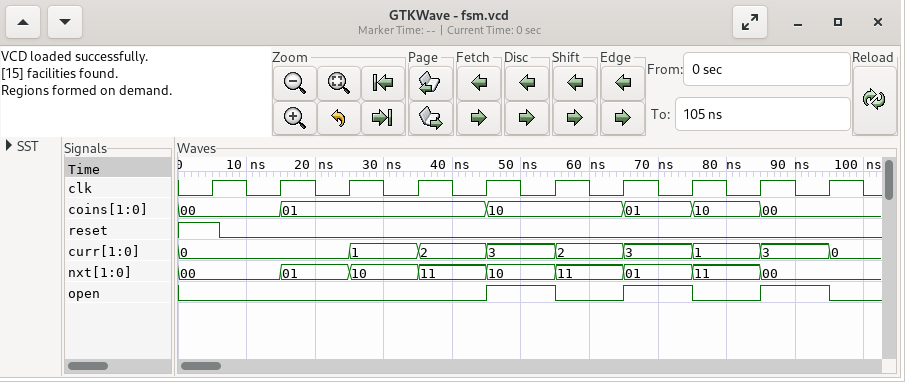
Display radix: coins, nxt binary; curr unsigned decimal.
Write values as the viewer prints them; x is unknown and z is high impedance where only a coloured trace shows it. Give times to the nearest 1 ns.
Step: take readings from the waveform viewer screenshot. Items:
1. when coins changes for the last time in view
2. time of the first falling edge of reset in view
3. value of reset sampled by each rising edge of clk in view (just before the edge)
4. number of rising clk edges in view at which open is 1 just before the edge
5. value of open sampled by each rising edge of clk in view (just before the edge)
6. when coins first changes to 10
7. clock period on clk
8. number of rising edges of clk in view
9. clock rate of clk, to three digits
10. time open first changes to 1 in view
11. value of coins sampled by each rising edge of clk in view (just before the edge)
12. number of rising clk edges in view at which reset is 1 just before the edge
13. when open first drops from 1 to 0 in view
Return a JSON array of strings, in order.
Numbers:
["85 ns", "6 ns", "1 0 0 0 0 0 0 0 0 0", "3", "0 0 0 0 0 1 0 1 0 1", "45 ns", "10 ns", "10", "100 MHz", "45 ns", "00, 00, 01, 01, 01, 10, 10, 01, 10, 00", "1", "55 ns"]
